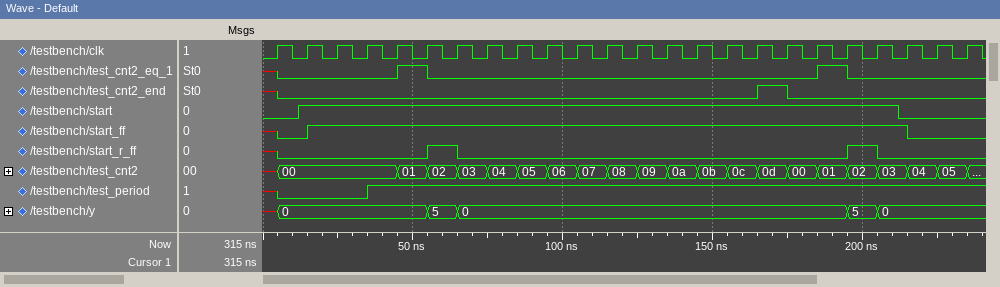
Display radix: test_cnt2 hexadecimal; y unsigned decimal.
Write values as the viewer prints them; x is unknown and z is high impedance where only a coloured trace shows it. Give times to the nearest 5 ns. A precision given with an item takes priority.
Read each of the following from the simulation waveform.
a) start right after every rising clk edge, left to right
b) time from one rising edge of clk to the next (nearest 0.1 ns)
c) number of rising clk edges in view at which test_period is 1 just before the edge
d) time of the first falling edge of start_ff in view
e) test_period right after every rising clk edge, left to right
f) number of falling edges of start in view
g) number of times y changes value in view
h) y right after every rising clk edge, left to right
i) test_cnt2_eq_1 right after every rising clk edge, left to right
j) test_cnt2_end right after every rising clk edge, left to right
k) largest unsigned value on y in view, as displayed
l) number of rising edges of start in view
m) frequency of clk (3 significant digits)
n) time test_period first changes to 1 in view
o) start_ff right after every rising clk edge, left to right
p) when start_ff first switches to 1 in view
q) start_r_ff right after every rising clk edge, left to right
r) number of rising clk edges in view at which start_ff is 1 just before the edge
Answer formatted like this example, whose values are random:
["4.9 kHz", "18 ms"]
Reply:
["0 1 1 1 1 1 1 1 1 1 1 1 1 1 1 1 1 1 1 1 1 0 0 0", "10 ns", "20", "215 ns", "0 0 0 1 1 1 1 1 1 1 1 1 1 1 1 1 1 1 1 1 1 1 1 1", "1", "5", "0, 0, 0, 0, 0, 5, 0, 0, 0, 0, 0, 0, 0, 0, 0, 0, 0, 0, 0, 5, 0, 0, 0, 0", "0 0 0 0 1 0 0 0 0 0 0 0 0 0 0 0 0 0 1 0 0 0 0 0", "0 0 0 0 0 0 0 0 0 0 0 0 0 0 0 0 1 0 0 0 0 0 0 0", "5", "1", "100 MHz", "35 ns", "0 1 1 1 1 1 1 1 1 1 1 1 1 1 1 1 1 1 1 1 1 0 0 0", "15 ns", "0 0 0 0 0 1 0 0 0 0 0 0 0 0 0 0 0 0 0 1 0 0 0 0", "20"]
